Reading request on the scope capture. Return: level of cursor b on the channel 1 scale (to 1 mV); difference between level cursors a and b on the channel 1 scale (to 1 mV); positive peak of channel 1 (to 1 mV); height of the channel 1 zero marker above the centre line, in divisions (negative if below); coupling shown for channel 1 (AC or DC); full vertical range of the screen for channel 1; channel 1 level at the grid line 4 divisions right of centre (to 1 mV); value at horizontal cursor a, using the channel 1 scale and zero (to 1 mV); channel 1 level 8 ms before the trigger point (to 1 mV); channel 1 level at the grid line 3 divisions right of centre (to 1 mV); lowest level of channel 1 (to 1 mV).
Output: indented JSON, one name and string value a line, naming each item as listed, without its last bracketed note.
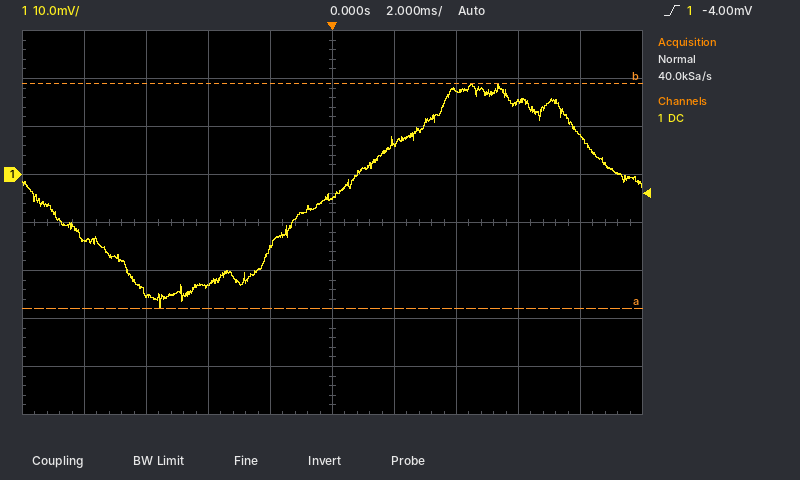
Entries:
{
  "level of cursor b on the channel 1 scale": "19 mV",
  "difference between level cursors a and b on the channel 1 scale": "47 mV",
  "positive peak of channel 1": "19 mV",
  "height of the channel 1 zero marker above the centre line, in divisions": "+1.0 div",
  "coupling shown for channel 1": "DC",
  "full vertical range of the screen for channel 1": "80 mV",
  "channel 1 level at the grid line 4 divisions right of centre": "8 mV",
  "value at horizontal cursor a, using the channel 1 scale and zero": "-28 mV",
  "channel 1 level 8 ms before the trigger point": "-14 mV",
  "channel 1 level at the grid line 3 divisions right of centre": "15 mV",
  "lowest level of channel 1": "-28 mV"
}
